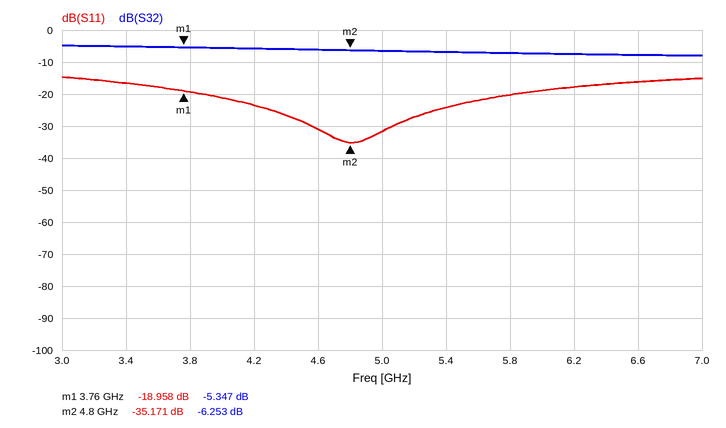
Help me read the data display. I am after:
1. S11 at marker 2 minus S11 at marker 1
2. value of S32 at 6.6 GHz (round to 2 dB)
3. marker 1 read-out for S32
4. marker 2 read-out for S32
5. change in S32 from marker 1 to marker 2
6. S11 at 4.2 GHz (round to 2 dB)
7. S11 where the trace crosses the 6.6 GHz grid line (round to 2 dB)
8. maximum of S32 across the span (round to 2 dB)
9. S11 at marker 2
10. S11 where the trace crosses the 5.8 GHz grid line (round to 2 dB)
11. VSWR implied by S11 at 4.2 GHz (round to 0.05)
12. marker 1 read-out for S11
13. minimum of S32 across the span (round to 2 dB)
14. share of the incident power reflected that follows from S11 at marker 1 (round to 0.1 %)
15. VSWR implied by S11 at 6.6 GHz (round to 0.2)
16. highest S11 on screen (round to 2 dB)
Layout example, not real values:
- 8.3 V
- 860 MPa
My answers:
- -16.213 dB
- -8 dB
- -5.347 dB
- -6.253 dB
- -0.906 dB
- -24 dB
- -16 dB
- -4 dB
- -35.171 dB
- -20 dB
- 1.15
- -18.958 dB
- -8 dB
- 1.3 %
- 1.4
- -14 dB
